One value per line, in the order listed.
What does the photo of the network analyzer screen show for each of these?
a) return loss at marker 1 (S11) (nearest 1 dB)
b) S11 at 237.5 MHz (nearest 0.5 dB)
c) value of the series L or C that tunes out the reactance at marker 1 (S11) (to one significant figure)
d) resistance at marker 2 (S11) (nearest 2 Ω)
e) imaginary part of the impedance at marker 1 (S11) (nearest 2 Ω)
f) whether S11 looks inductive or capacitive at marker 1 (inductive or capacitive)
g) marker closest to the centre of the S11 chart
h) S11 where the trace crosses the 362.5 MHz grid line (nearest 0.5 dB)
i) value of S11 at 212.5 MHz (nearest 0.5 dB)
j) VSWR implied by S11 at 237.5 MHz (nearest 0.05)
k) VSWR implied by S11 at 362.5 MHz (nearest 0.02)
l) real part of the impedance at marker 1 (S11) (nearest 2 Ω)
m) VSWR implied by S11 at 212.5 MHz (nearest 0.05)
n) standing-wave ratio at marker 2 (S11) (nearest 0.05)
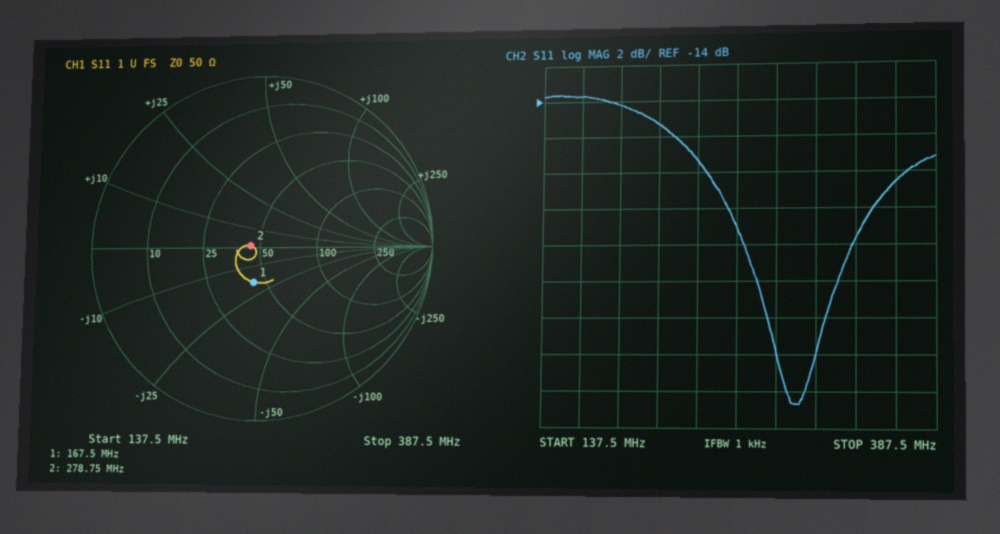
14 dB
-17.5 dB
20 nH
44 Ω
-18 Ω
capacitive
marker 2
-18.5 dB
-15.5 dB
1.30
1.26
44 Ω
1.40
1.10
